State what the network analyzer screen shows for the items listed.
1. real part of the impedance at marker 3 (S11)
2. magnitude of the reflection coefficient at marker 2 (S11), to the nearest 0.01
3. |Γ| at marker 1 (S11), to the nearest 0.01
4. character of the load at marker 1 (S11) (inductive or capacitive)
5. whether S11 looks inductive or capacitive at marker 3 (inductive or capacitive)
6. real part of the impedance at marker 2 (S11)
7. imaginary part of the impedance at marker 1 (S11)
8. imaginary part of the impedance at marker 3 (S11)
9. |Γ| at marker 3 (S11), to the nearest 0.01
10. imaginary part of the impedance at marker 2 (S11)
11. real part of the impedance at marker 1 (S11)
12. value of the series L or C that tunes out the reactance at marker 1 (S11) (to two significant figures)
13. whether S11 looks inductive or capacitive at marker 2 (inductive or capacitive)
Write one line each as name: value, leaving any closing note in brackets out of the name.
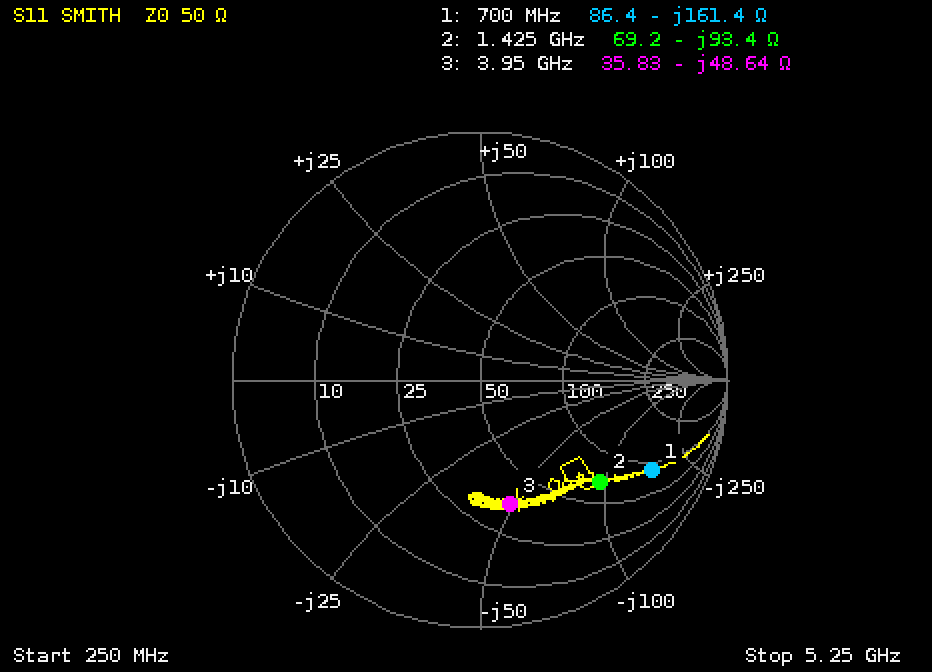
real part of the impedance at marker 3: 35.83 Ω
magnitude of the reflection coefficient at marker 2 (S11), to the nearest 0.01: 0.63
|Γ| at marker 1 (S11), to the nearest 0.01: 0.78
character of the load at marker 1 (S11): capacitive
whether S11 looks inductive or capacitive at marker 3: capacitive
real part of the impedance at marker 2: 69.2 Ω
imaginary part of the impedance at marker 1: -161.4 Ω
imaginary part of the impedance at marker 3: -48.64 Ω
|Γ| at marker 3 (S11), to the nearest 0.01: 0.51
imaginary part of the impedance at marker 2: -93.4 Ω
real part of the impedance at marker 1: 86.4 Ω
value of the series L or C that tunes out the reactance at marker 1 (S11): 37 nH
whether S11 looks inductive or capacitive at marker 2: capacitive
